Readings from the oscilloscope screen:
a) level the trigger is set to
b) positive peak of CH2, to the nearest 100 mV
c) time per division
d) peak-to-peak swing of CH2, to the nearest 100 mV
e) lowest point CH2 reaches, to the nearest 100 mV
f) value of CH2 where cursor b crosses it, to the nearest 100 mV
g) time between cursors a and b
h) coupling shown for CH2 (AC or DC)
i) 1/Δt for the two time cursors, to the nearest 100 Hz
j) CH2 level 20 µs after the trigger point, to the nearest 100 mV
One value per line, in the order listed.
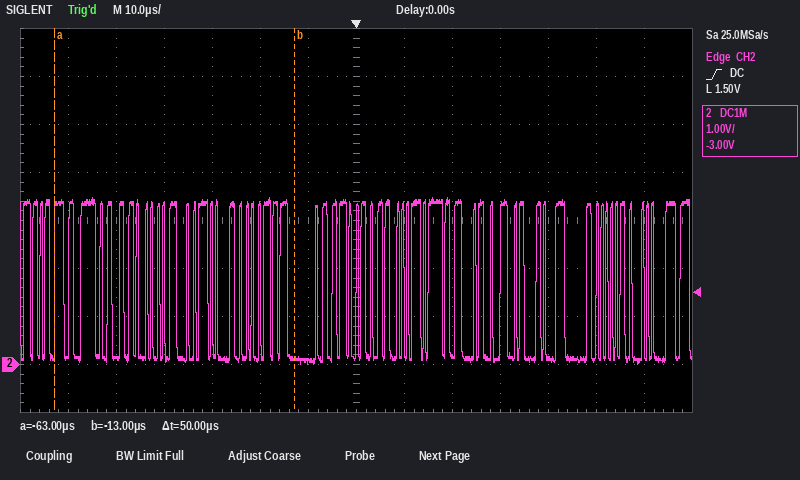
1.50 V
3.5 V
10 µs
3.5 V
0.0 V
100 mV
50 µs
DC
20.0 kHz
200 mV
